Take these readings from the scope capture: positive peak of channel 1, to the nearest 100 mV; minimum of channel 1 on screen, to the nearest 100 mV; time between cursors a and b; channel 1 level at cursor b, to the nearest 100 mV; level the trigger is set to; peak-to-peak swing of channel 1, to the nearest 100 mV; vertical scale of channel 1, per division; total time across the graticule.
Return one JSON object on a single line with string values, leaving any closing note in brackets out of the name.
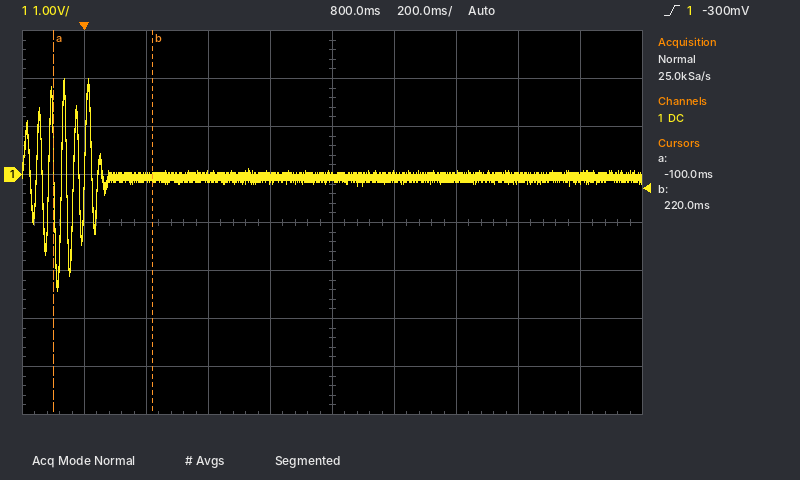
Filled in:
{"positive peak of channel 1, to the nearest 100 mV": "2.0 V", "minimum of channel 1 on screen, to the nearest 100 mV": "-2.4 V", "time between cursors a and b": "320 ms", "channel 1 level at cursor b, to the nearest 100 mV": "-100 mV", "level the trigger is set to": "-300 mV", "peak-to-peak swing of channel 1, to the nearest 100 mV": "4.4 V", "vertical scale of channel 1, per division": "1 V", "total time across the graticule": "2 s"}
